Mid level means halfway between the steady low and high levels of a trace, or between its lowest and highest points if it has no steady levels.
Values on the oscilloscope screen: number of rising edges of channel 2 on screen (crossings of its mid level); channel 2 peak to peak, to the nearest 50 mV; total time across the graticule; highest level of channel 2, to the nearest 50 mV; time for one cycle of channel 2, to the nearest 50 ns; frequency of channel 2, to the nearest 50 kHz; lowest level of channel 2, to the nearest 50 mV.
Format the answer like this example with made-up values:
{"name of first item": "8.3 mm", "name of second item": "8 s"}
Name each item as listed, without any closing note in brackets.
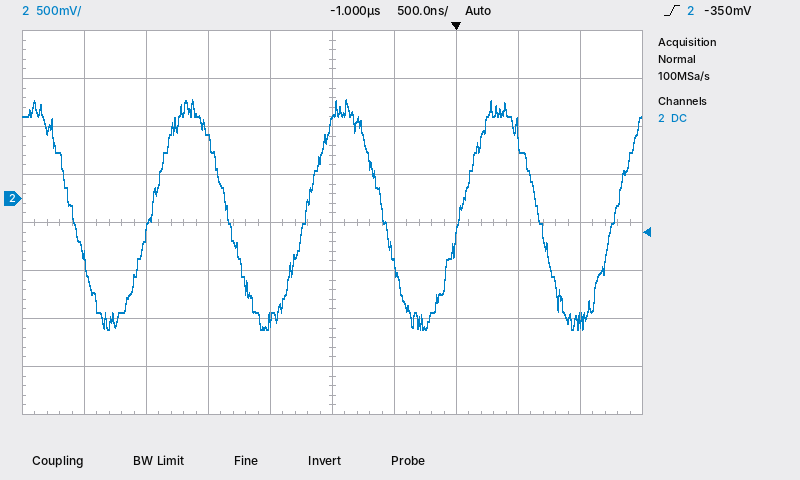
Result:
{"number of rising edges of channel 2 on screen": "4", "channel 2 peak to peak, to the nearest 50 mV": "2.40 V", "total time across the graticule": "5 µs", "highest level of channel 2, to the nearest 50 mV": "1.05 V", "time for one cycle of channel 2, to the nearest 50 ns": "1.25 µs", "frequency of channel 2, to the nearest 50 kHz": "800 kHz", "lowest level of channel 2, to the nearest 50 mV": "-1.35 V"}
